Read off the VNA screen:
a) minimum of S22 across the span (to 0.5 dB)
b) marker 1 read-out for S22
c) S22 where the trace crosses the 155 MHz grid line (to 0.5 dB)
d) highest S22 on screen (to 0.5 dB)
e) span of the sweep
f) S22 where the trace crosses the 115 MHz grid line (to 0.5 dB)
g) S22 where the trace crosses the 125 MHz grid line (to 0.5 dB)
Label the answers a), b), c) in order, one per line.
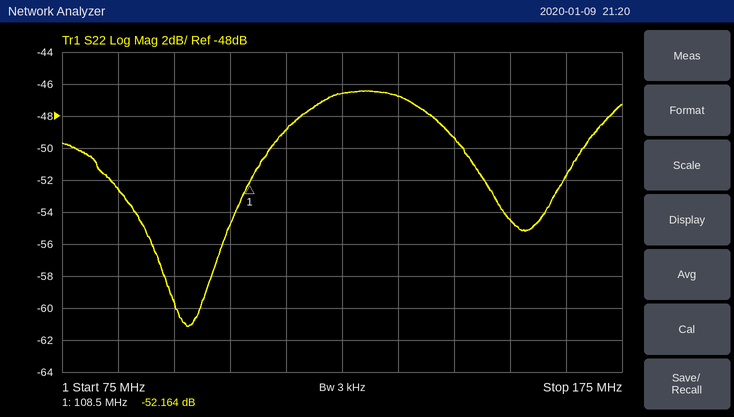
a) -61.0 dB
b) -52.164 dB
c) -54.5 dB
d) -46.5 dB
e) 100 MHz
f) -49.0 dB
g) -46.5 dB
